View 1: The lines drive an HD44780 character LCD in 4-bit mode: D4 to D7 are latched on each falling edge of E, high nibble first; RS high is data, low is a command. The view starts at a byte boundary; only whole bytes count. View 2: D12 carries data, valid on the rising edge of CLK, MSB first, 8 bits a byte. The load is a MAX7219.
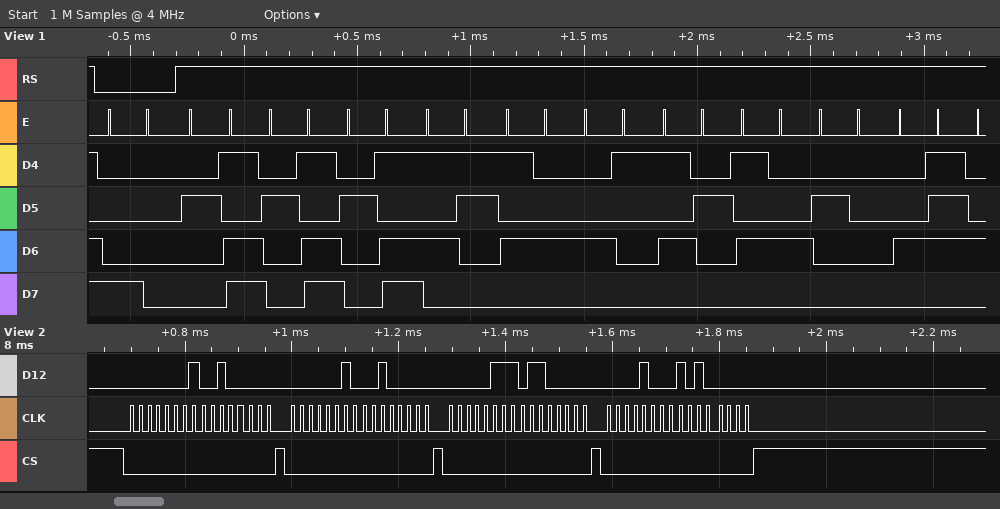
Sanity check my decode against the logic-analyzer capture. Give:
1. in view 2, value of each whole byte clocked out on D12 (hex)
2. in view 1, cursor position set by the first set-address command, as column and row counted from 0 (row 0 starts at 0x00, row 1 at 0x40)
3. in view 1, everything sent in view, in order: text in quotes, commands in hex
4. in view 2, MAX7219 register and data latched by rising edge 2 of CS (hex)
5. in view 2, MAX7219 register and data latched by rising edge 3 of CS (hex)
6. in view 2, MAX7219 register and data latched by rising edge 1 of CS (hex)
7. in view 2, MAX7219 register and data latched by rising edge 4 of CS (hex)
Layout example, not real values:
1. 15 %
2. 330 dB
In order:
1. 01 20 02 20 07 60 08 A0
2. column 0, row 0
3. 0x80 "---START G"
4. register 0x2, data 0x20
5. register 0x7, data 0x60
6. register 0x1, data 0x20
7. register 0x8, data 0xA0
